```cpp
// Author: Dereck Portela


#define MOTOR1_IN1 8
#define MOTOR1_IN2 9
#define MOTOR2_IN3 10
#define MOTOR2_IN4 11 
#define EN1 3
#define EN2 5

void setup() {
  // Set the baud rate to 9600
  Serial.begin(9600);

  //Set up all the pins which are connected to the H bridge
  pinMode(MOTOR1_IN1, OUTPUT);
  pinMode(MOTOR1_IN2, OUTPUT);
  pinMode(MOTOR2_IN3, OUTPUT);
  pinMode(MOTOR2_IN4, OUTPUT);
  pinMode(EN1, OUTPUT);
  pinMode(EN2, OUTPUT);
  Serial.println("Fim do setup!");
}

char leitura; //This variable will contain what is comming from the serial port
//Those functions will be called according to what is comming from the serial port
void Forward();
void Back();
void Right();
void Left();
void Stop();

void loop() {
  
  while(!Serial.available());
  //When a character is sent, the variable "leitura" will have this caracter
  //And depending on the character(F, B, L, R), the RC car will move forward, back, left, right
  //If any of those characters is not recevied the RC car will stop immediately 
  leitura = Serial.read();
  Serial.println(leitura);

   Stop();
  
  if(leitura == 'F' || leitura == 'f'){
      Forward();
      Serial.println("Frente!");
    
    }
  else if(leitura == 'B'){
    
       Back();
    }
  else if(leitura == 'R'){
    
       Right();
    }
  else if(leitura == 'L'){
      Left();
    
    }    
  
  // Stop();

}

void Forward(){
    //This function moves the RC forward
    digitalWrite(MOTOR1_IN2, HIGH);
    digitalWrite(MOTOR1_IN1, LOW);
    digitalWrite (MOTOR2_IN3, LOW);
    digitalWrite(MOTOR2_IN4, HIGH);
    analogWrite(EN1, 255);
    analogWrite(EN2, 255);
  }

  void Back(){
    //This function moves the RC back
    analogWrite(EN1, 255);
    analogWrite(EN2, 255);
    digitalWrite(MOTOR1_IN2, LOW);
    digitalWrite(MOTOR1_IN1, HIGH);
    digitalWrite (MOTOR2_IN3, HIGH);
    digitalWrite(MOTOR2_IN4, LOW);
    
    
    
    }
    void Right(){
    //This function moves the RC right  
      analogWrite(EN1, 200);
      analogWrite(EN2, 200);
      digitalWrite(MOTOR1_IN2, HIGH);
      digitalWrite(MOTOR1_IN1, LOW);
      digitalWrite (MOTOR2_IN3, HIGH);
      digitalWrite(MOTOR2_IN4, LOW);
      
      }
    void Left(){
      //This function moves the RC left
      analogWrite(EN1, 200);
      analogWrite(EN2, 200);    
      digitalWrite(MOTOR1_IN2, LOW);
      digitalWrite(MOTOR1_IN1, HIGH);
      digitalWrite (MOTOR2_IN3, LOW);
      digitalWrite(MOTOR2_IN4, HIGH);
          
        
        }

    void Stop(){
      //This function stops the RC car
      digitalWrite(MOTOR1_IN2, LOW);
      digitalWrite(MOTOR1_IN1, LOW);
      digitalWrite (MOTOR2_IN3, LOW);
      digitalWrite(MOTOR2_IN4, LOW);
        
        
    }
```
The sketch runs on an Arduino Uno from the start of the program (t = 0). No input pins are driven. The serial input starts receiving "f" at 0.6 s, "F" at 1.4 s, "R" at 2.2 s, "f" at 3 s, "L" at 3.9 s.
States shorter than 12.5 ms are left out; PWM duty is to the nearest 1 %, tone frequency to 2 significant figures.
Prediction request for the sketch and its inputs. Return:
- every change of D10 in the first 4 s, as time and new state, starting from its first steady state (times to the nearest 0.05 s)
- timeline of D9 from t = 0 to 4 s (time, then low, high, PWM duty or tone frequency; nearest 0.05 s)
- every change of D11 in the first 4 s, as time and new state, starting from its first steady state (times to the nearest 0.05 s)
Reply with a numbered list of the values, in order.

1. 0 s low; 2.2 s high; 3 s low
2. 0 s low; 0.6 s high; 3.9 s low
3. 0 s low; 0.6 s high; 2.2 s low; 3 s high
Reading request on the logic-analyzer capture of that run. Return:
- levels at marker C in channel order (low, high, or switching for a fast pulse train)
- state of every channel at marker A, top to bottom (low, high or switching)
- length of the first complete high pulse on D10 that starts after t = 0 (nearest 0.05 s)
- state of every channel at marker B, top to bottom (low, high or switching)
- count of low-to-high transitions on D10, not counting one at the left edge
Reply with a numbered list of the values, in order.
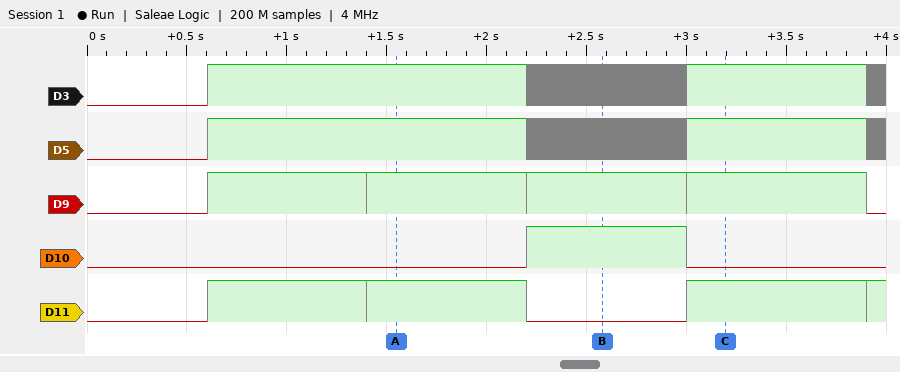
1. D3 high, D5 high, D9 high, D10 low, D11 high
2. D3 high, D5 high, D9 high, D10 low, D11 high
3. 0.80 s
4. D3 switching, D5 switching, D9 high, D10 high, D11 low
5. 1
